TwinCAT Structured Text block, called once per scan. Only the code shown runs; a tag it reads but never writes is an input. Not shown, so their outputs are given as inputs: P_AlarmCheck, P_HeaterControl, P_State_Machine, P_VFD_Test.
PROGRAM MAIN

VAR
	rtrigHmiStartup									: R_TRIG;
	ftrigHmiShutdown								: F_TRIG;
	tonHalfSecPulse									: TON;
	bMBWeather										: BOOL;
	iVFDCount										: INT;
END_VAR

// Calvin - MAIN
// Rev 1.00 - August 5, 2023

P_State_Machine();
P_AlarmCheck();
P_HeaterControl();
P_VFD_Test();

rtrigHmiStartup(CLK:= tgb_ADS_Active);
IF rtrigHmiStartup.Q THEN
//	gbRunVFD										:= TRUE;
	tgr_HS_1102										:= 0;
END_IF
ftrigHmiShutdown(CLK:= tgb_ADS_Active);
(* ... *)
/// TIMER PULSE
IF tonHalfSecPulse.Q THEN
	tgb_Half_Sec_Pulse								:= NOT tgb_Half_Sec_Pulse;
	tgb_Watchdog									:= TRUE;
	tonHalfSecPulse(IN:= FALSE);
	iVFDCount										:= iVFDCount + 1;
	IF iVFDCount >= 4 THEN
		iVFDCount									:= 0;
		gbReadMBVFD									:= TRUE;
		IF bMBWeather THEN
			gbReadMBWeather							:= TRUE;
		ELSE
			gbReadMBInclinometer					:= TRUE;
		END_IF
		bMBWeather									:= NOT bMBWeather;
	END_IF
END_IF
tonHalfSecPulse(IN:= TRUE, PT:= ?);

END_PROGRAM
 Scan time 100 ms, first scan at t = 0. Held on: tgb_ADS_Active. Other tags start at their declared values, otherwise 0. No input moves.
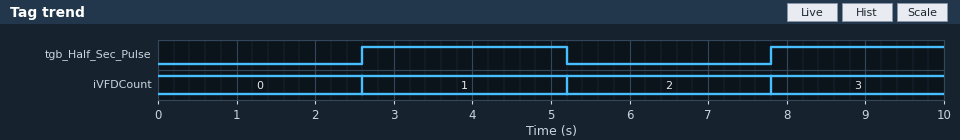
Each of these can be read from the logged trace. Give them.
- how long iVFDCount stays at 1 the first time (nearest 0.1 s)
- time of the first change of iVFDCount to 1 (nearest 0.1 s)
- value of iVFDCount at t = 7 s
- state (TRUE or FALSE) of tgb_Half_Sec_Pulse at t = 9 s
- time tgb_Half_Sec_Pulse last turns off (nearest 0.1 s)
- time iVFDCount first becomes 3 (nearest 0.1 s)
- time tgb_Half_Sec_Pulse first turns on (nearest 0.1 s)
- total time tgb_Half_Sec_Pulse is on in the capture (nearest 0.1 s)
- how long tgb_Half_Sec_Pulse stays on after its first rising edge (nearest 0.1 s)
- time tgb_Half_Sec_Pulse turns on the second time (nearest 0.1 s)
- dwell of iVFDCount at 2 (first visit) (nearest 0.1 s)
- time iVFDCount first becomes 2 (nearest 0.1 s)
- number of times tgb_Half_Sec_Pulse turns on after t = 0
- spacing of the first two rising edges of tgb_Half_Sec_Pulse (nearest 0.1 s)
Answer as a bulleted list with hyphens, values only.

- 2.6 s
- 2.6 s
- 2
- TRUE
- 5.2 s
- 7.8 s
- 2.6 s
- 4.8 s
- 2.6 s
- 7.8 s
- 2.6 s
- 5.2 s
- 2
- 5.2 s
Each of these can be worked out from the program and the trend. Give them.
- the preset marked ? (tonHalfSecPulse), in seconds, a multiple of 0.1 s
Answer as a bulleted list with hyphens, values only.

- 2.5 s
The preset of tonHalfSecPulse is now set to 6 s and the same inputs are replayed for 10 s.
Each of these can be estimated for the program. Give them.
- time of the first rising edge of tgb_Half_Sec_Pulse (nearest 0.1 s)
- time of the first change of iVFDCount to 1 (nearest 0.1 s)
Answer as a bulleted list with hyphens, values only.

- 6.1 s
- 6.1 s
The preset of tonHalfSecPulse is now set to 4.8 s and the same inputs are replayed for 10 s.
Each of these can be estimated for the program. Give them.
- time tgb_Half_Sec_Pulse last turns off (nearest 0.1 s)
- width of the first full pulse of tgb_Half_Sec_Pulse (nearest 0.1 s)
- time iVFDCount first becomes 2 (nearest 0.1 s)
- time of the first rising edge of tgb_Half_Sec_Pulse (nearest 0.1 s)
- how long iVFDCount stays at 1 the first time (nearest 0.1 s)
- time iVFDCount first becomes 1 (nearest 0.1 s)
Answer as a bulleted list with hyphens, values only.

- 9.8 s
- 4.9 s
- 9.8 s
- 4.9 s
- 4.9 s
- 4.9 s
